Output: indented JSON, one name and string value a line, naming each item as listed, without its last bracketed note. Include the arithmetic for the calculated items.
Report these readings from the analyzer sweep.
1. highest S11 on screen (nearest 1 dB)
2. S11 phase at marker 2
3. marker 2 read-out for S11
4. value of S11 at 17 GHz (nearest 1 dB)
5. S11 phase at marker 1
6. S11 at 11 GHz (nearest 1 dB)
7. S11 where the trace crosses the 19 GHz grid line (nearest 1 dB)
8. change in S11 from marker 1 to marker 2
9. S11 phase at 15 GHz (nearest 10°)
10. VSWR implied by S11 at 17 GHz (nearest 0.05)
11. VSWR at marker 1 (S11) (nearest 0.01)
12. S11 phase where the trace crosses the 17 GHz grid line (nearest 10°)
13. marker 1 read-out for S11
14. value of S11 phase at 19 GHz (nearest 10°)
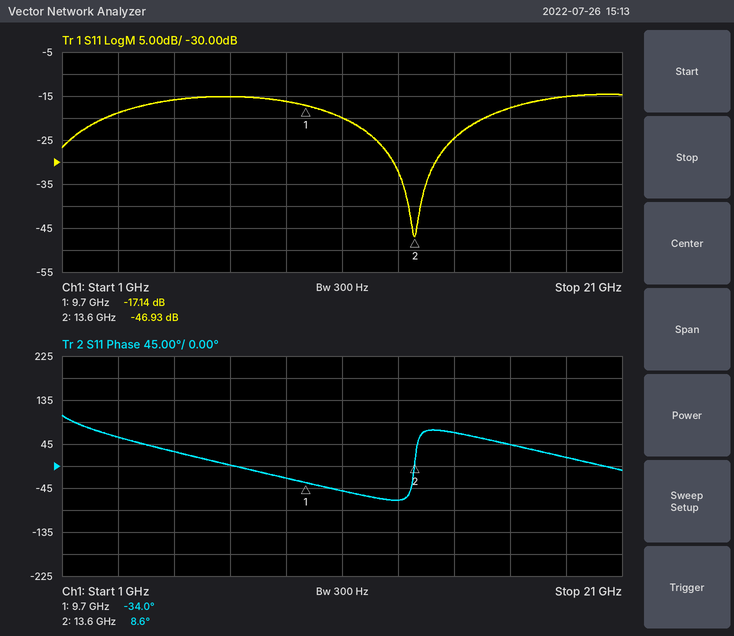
{
  "highest S11 on screen": "-15 dB",
  "S11 phase at marker 2": "8.6°",
  "marker 2 read-out for S11": "-46.93 dB",
  "value of S11 at 17 GHz": "-18 dB",
  "S11 phase at marker 1": "-34.0°",
  "S11 at 11 GHz": "-20 dB",
  "S11 where the trace crosses the 19 GHz grid line": "-15 dB",
  "change in S11 from marker 1 to marker 2": "-46.93 − (-17.14) = -29.79 dB",
  "S11 phase at 15 GHz": "70°",
  "VSWR implied by S11 at 17 GHz": "|Γ| = 10^(-18/20) = 0.1259; VSWR = (1 + 0.1259)/(1 − 0.1259) ≈ 1.29, so 1.30 to the nearest 0.05",
  "VSWR at marker 1 (S11)": "(1 + 0.1390)/(1 − 0.1390) ≈ 1.32",
  "S11 phase where the trace crosses the 17 GHz grid line": "40°",
  "marker 1 read-out for S11": "-17.14 dB",
  "value of S11 phase at 19 GHz": "20°"
}
